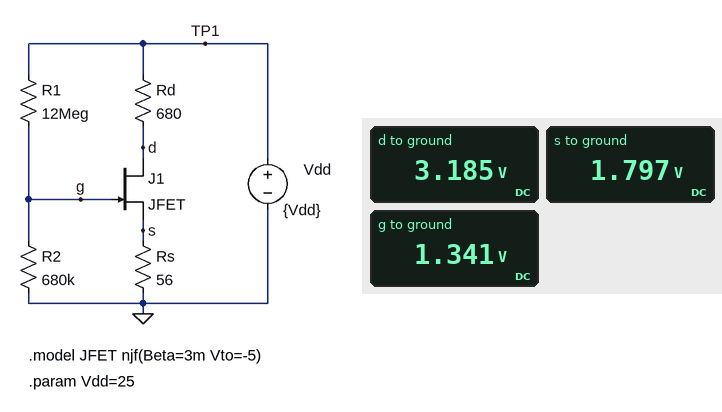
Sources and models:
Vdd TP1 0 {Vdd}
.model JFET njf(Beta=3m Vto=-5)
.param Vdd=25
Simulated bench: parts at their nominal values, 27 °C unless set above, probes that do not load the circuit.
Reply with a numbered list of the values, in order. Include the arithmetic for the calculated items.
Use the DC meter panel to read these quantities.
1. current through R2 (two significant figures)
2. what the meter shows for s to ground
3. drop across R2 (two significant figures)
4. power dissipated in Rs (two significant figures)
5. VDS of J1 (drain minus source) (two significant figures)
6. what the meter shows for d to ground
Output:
1. (1.341 V) / 680 kΩ = 2.0 µA
2. 1.797 V
3. 1.341 V = 1.3 V
4. (1.797 V)^2 / 56 Ω = 58 mW
5. 3.185 V - 1.797 V = 1.4 V
6. 3.185 V
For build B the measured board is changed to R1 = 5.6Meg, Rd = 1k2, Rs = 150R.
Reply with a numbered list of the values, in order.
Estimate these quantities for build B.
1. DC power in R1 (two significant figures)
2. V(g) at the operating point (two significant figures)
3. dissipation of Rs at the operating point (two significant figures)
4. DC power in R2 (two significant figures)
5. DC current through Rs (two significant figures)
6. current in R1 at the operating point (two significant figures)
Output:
1. 89 µW
2. 2.7 V
3. 49 mW
4. 11 µW
5. 18 mA
6. 4.0 µA
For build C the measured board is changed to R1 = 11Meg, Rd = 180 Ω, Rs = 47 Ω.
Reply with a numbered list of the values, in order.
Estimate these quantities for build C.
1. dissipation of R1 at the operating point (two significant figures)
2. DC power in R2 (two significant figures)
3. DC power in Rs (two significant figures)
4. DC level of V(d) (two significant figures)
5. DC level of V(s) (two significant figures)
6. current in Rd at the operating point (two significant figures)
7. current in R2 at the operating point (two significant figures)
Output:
1. 50 µW
2. 3.1 µW
3. 120 mW
4. 16 V
5. 2.4 V
6. 50 mA
7. 2.1 µA
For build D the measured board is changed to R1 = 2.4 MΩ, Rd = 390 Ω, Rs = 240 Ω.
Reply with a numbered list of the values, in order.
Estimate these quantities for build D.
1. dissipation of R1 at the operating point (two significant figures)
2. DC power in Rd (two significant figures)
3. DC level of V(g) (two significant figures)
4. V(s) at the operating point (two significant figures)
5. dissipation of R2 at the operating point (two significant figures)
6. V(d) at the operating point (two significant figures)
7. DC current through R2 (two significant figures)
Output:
1. 160 µW
2. 360 mW
3. 5.5 V
4. 7.3 V
5. 45 µW
6. 13 V
7. 8.1 µA
